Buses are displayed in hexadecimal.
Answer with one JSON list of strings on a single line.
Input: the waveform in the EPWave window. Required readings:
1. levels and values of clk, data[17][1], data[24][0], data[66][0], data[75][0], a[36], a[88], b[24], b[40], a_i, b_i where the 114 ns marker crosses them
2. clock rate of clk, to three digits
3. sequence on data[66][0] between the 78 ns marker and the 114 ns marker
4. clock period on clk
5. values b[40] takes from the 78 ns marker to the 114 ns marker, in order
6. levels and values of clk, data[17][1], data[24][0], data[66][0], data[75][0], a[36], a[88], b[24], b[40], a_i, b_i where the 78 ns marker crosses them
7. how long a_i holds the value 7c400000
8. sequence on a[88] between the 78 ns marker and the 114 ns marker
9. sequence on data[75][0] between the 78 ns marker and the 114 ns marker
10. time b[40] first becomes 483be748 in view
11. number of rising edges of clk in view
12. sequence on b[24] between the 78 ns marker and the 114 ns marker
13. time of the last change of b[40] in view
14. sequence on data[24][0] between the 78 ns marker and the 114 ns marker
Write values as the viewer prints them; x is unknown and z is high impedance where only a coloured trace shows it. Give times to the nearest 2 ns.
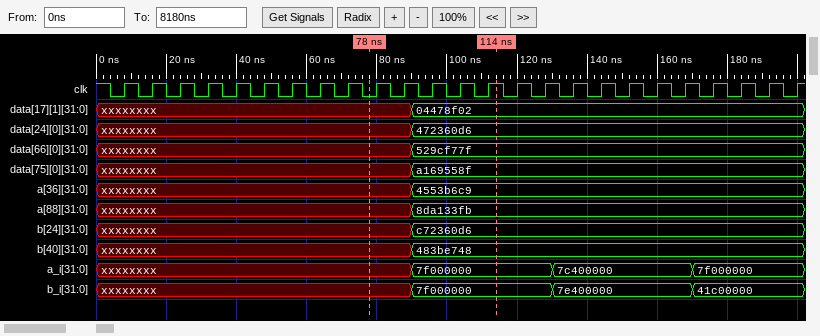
["clk=1, data[17][1]=04478f02, data[24][0]=472360d6, data[66][0]=529cf77f, data[75][0]=a169558f, a[36]=4553b6c9, a[88]=8da133fb, b[24]=c72360d6, b[40]=483be748, a_i=7f000000, b_i=7f000000", "125 MHz", "xxxxxxxx, 529cf77f", "8 ns", "xxxxxxxx, 483be748", "clk=0, data[17][1]=xxxxxxxx, data[24][0]=xxxxxxxx, data[66][0]=xxxxxxxx, data[75][0]=xxxxxxxx, a[36]=xxxxxxxx, a[88]=xxxxxxxx, b[24]=xxxxxxxx, b[40]=xxxxxxxx, a_i=xxxxxxxx, b_i=xxxxxxxx", "40 ns", "xxxxxxxx, 8da133fb", "xxxxxxxx, a169558f", "90 ns", "25", "xxxxxxxx, c72360d6", "90 ns", "xxxxxxxx, 472360d6"]
